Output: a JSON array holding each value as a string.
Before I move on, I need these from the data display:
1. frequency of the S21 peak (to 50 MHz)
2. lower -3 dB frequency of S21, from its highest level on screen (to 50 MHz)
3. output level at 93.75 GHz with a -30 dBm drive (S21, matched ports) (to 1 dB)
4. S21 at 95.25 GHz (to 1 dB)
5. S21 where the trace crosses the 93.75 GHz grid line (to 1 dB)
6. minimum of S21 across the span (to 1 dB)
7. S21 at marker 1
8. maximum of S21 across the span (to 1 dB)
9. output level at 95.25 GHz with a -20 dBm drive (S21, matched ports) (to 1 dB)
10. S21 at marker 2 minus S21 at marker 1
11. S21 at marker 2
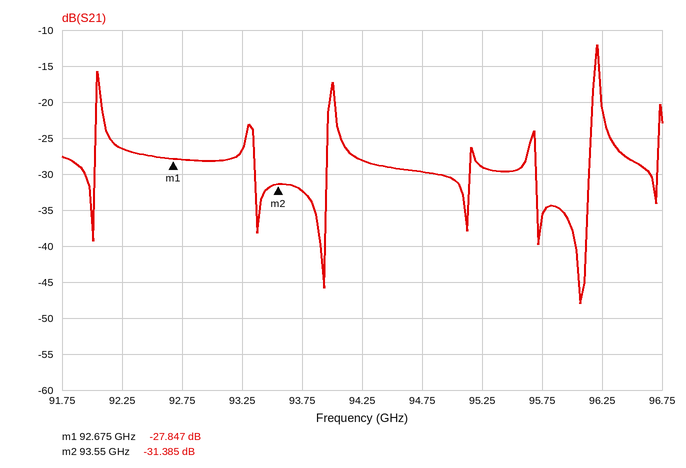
["96.20 GHz", "96.20 GHz", "-62 dBm", "-29 dB", "-32 dB", "-48 dB", "-27.847 dB", "-12 dB", "-49 dBm", "-3.538 dB", "-31.385 dB"]
